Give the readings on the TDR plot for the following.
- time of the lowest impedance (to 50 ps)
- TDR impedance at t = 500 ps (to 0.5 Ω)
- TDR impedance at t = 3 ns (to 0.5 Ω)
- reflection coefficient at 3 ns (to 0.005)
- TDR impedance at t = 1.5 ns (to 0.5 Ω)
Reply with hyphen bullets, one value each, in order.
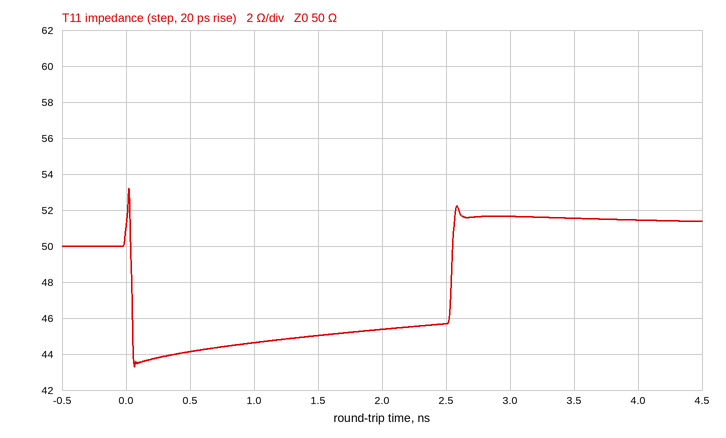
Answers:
- 50 ps
- 44.0 Ω
- 51.5 Ω
- +0.015
- 45.0 Ω
